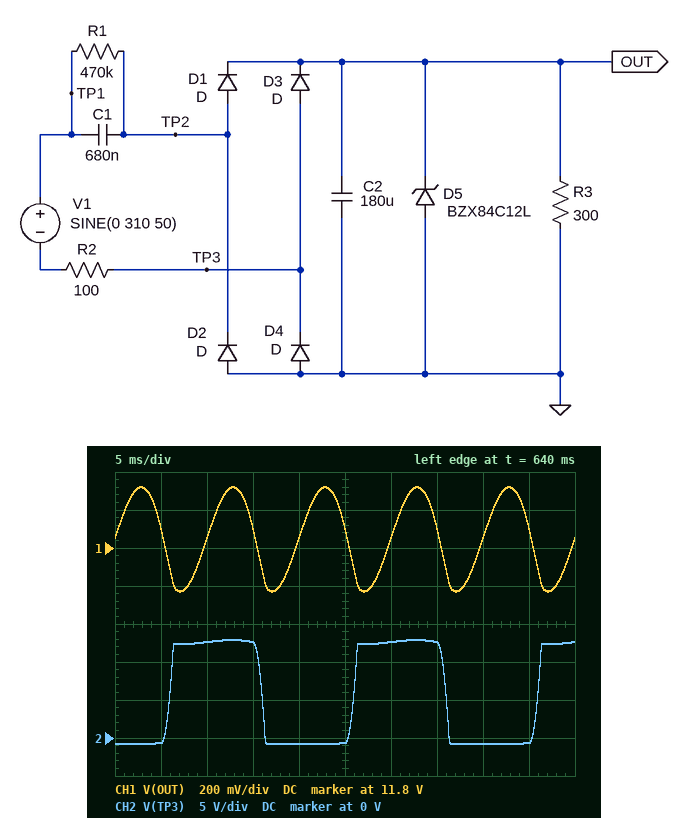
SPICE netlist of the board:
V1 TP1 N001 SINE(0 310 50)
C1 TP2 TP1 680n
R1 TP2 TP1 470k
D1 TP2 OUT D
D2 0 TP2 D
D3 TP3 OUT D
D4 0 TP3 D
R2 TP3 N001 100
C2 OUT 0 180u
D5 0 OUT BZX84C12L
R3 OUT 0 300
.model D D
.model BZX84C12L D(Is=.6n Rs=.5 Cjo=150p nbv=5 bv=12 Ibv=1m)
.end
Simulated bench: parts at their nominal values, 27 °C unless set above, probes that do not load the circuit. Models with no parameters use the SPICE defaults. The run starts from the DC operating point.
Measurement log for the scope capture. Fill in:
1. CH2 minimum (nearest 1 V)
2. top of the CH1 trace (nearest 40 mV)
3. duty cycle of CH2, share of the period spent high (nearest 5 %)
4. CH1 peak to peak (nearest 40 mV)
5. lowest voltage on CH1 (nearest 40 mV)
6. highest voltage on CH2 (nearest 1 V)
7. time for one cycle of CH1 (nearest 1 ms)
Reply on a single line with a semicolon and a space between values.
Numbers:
-1 V; 12.12 V; 50 %; 560 mV; 11.56 V; 13 V; 10 ms
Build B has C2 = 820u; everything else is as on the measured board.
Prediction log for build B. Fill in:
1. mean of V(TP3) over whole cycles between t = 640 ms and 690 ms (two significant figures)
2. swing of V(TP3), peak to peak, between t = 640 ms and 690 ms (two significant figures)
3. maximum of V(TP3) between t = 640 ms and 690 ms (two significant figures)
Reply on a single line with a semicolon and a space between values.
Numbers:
5.7 V; 13 V; 12 V
